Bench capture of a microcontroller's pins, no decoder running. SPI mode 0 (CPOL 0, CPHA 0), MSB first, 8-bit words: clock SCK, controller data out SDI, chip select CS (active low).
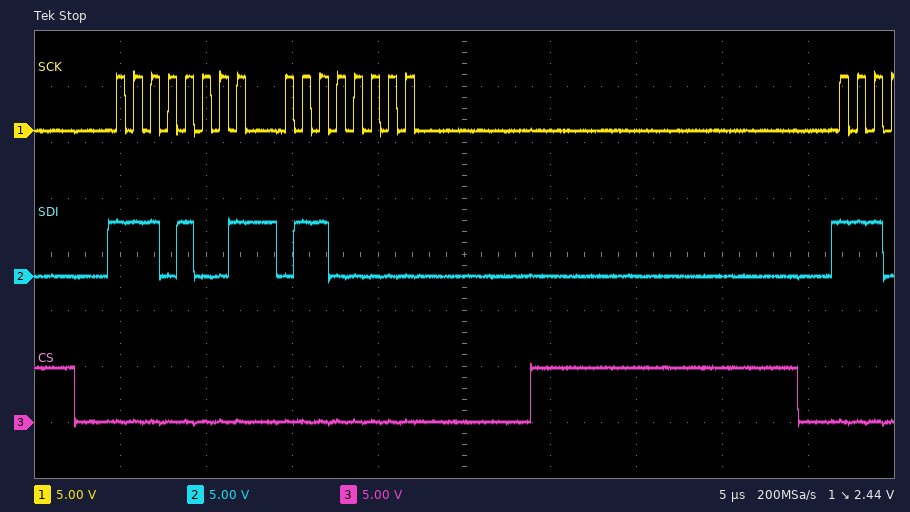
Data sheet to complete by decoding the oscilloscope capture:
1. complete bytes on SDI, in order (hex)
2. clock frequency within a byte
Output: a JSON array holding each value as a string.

["0xE9 0x60", "1 MHz"]
